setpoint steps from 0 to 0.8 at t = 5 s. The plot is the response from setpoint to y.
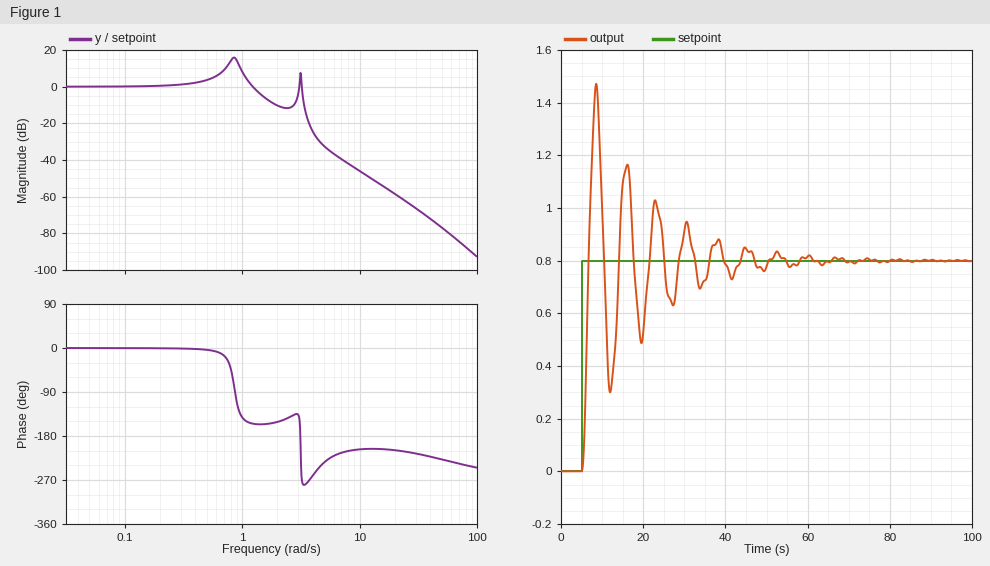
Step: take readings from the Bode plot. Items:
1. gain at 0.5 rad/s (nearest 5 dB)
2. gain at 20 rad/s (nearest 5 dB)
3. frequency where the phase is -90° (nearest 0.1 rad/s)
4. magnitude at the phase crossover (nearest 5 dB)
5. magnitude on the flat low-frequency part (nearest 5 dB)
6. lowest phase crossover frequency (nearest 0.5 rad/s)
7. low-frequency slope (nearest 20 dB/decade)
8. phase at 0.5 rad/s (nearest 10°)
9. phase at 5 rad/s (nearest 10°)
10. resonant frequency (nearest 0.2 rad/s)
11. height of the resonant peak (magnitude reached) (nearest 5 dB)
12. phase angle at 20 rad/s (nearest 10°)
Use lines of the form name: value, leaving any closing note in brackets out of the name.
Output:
gain at 0.5 rad/s: 5 dB
gain at 20 rad/s: -60 dB
frequency where the phase is -90°: 0.9 rad/s
magnitude at the phase crossover: 5 dB
magnitude on the flat low-frequency part: 0 dB
lowest phase crossover frequency: 3.0 rad/s
low-frequency slope: 0 dB/decade
phase at 0.5 rad/s: 0°
phase at 5 rad/s: -230°
resonant frequency: 0.8 rad/s
height of the resonant peak (magnitude reached): 15 dB
phase angle at 20 rad/s: -210°
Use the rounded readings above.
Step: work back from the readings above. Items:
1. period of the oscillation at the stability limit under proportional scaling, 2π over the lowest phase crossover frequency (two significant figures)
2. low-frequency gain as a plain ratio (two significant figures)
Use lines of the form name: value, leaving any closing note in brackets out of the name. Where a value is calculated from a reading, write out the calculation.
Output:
period of the oscillation at the stability limit under proportional scaling, 2π over the lowest phase crossover frequency: 2π / 3 = 2.1 s
low-frequency gain as a plain ratio: 10^(0 / 20) = 1.0
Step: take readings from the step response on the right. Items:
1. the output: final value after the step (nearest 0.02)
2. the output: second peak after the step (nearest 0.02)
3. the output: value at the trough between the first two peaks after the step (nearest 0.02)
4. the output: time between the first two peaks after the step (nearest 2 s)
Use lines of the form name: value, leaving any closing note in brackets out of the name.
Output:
the output: final value after the step: 0.80
the output: second peak after the step: 1.16
the output: value at the trough between the first two peaks after the step: 0.30
the output: time between the first two peaks after the step: 8 s
